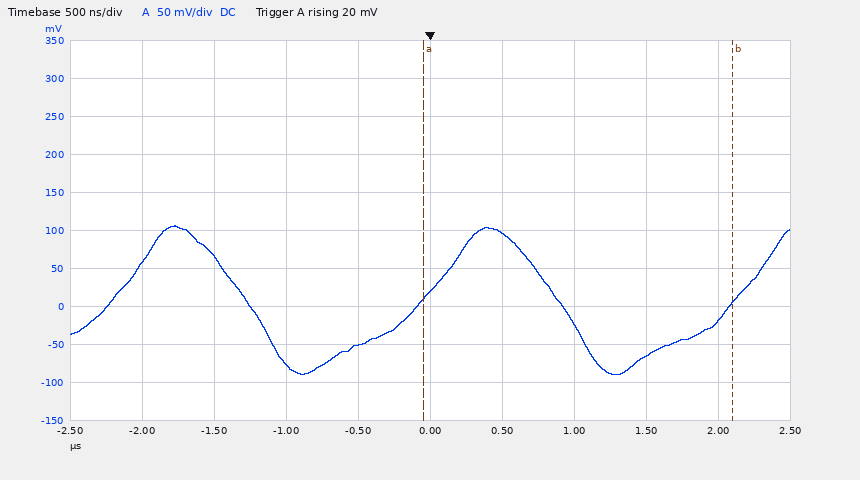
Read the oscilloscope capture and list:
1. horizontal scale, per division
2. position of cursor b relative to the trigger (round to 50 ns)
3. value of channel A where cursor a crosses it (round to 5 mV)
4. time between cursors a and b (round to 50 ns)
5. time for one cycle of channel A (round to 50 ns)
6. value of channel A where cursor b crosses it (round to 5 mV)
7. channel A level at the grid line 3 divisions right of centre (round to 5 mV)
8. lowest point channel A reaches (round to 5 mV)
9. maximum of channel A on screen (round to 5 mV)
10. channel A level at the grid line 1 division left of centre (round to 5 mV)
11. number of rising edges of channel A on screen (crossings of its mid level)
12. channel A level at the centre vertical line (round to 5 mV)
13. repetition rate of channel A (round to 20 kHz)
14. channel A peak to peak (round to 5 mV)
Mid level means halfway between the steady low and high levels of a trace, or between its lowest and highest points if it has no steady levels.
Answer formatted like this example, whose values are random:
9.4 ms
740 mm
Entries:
500 ns
+2.10 µs
10 mV
2.15 µs
2.15 µs
5 mV
-65 mV
-90 mV
105 mV
-50 mV
3
20 mV
460 kHz
195 mV
